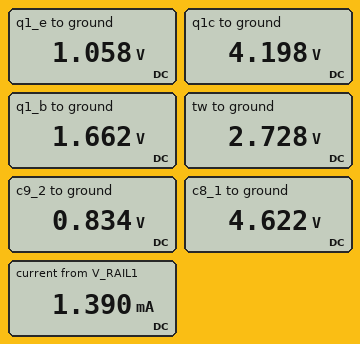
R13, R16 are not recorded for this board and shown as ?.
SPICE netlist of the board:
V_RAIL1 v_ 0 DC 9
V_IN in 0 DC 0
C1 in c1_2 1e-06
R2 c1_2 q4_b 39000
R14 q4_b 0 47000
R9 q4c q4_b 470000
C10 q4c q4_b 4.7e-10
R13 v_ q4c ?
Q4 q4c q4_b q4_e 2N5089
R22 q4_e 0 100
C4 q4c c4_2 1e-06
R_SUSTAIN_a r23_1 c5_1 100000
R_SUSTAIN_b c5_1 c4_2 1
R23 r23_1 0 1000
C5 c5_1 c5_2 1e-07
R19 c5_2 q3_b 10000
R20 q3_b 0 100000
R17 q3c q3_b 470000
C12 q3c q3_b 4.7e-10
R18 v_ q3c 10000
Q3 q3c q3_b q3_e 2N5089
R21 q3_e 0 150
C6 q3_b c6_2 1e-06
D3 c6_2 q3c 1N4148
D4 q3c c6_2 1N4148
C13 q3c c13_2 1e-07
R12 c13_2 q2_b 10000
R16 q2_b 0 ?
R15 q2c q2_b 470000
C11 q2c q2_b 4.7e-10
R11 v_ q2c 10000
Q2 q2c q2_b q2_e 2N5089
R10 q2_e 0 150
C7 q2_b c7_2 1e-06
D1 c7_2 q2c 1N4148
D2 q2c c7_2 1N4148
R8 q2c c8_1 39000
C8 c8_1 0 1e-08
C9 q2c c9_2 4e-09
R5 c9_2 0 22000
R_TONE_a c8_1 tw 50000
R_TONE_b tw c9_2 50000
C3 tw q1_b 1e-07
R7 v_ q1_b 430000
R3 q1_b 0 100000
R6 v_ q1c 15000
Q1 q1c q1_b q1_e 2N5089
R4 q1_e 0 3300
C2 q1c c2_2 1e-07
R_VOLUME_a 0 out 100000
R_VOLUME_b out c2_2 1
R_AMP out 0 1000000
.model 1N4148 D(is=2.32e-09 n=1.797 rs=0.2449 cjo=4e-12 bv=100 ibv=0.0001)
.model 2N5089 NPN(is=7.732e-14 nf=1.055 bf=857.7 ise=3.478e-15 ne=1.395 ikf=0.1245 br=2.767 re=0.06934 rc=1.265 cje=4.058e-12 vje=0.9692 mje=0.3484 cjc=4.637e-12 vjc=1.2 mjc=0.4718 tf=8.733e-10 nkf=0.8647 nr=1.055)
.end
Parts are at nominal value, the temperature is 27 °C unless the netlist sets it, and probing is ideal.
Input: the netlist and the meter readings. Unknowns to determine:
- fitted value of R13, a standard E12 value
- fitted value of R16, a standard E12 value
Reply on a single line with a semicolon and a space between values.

6.8 kΩ; 56 kΩ
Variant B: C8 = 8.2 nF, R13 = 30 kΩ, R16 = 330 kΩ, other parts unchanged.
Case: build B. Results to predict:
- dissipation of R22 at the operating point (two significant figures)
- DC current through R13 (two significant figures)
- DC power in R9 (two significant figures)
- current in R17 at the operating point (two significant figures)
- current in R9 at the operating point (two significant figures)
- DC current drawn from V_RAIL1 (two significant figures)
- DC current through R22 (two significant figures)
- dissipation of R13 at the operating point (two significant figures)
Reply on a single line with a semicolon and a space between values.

580 nW; 88 µA; 71 µW; 7.5 µA; 12 µA; 1.6 mA; 76 µA; 230 µW
